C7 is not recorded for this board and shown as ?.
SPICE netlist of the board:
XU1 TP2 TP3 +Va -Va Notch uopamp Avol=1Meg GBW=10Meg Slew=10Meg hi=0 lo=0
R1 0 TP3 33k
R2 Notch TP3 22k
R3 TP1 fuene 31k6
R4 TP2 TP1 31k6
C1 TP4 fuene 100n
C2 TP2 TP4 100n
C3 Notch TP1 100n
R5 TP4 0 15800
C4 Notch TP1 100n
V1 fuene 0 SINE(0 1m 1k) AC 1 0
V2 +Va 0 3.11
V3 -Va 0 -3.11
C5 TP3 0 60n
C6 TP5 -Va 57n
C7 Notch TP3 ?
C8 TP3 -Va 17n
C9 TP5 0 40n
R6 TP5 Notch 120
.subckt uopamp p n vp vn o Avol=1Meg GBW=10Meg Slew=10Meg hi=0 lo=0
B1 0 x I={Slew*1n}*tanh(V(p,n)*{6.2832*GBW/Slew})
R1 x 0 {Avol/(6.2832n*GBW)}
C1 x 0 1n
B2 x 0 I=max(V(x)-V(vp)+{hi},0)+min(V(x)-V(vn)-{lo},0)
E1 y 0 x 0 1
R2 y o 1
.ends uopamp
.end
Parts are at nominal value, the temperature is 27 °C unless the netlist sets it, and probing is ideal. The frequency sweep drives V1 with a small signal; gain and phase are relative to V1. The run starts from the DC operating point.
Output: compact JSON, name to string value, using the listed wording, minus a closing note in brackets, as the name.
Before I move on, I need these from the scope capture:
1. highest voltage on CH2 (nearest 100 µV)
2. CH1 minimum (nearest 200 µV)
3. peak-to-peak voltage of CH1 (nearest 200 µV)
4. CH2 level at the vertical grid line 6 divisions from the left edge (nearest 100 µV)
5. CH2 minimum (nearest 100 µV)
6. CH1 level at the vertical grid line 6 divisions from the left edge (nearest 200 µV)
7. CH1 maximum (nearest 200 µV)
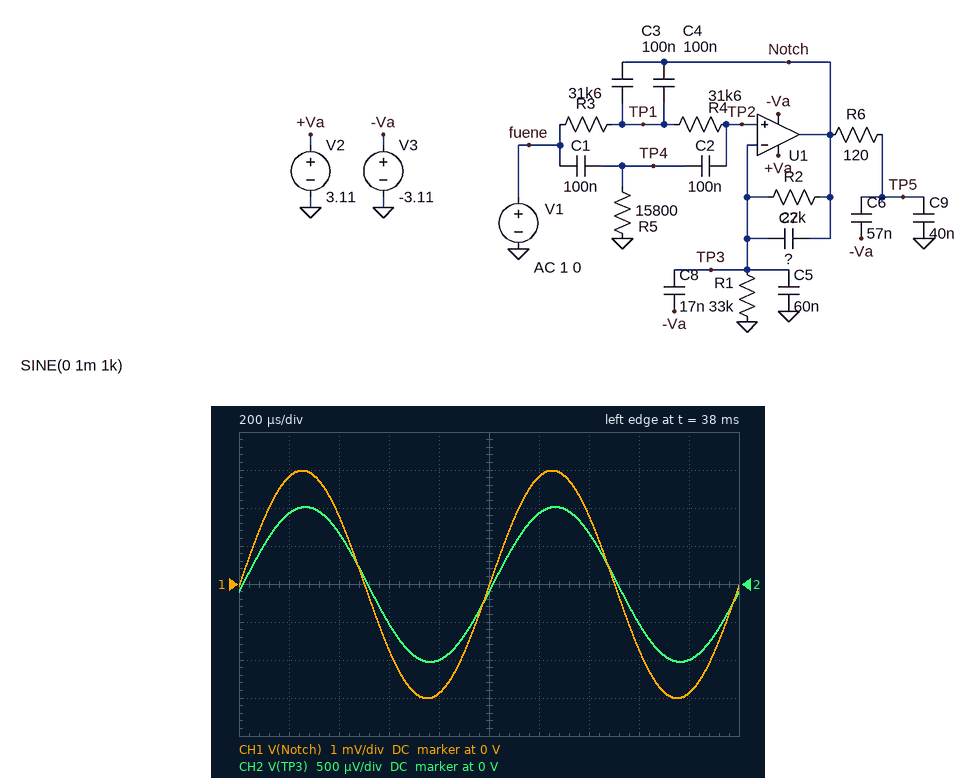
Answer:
{"highest voltage on CH2": "1.0 mV", "CH1 minimum": "-3.0 mV", "peak-to-peak voltage of CH1": "6.0 mV", "CH2 level at the vertical grid line 6 divisions from the left edge": "900 µV", "CH2 minimum": "-1.0 mV", "CH1 level at the vertical grid line 6 divisions from the left edge": "2.8 mV", "CH1 maximum": "3.0 mV"}
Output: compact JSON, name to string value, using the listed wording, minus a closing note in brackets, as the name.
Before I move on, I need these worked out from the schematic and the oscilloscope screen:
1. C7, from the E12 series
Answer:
{"C7, from the E12 series": "39 nF"}
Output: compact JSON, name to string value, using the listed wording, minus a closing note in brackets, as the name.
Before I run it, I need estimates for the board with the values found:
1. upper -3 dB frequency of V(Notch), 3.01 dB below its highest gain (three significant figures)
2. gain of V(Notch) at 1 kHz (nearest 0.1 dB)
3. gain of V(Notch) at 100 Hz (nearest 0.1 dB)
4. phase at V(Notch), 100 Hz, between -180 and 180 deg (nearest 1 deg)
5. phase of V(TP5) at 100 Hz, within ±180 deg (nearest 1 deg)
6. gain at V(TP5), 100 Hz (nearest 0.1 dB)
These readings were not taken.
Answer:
{"upper -3 dB frequency of V(Notch), 3.01 dB below its highest gain": "106 Hz", "gain of V(Notch) at 1 kHz": "9.5 dB", "gain of V(Notch) at 100 Hz": "17.6 dB", "phase at V(Notch), 100 Hz, between -180 and 180 deg": "27 deg", "phase of V(TP5) at 100 Hz, within ±180 deg": "26 deg", "gain at V(TP5), 100 Hz": "17.6 dB"}
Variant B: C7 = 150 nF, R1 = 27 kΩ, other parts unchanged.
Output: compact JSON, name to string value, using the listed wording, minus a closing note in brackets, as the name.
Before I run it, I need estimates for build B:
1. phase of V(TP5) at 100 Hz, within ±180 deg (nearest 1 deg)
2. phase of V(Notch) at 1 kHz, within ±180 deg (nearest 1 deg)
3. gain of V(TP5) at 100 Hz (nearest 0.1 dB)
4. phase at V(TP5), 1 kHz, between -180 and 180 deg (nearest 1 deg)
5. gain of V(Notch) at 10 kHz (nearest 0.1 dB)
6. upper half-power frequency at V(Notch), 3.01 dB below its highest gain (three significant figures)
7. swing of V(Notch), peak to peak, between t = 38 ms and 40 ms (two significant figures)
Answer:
{"phase of V(TP5) at 100 Hz, within ±180 deg": "22 deg", "phase of V(Notch) at 1 kHz, within ±180 deg": "2 deg", "gain of V(TP5) at 100 Hz": "1.7 dB", "phase at V(TP5), 1 kHz, between -180 and 180 deg": "-2 deg", "gain of V(Notch) at 10 kHz": "3.6 dB", "upper half-power frequency at V(Notch), 3.01 dB below its highest gain": "5.40 MHz", "swing of V(Notch), peak to peak, between t = 38 ms and 40 ms": "3.0 mV"}
